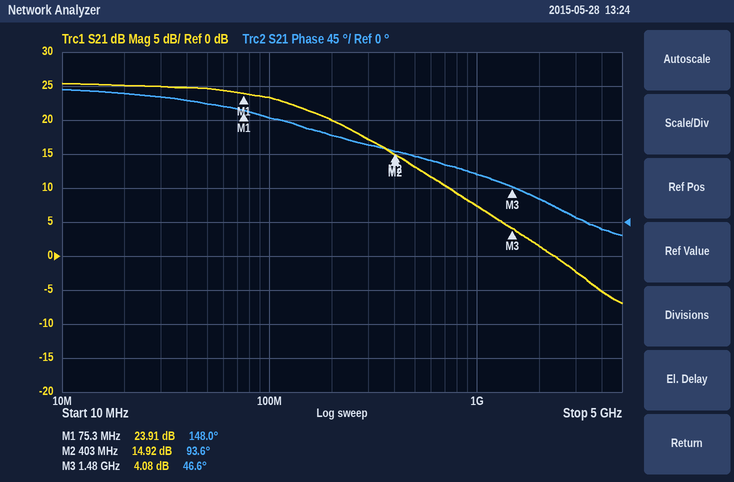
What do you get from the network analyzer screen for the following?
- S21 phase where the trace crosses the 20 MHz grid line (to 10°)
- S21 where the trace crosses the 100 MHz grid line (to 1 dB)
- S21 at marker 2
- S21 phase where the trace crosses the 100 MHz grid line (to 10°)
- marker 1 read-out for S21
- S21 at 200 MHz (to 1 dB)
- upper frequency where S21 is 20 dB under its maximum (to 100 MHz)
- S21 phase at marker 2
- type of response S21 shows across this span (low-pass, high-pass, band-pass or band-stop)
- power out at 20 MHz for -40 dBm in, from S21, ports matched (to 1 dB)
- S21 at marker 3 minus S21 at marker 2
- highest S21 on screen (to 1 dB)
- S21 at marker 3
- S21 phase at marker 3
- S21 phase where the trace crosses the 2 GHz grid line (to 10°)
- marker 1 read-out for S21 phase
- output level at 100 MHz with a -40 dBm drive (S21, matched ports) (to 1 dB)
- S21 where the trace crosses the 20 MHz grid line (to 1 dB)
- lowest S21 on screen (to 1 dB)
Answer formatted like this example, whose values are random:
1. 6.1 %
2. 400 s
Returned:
1. 170°
2. 23 dB
3. 14.92 dB
4. 140°
5. 23.91 dB
6. 20 dB
7. 1.3 GHz
8. 93.6°
9. low-pass
10. -15 dBm
11. -10.84 dB
12. 25 dB
13. 4.08 dB
14. 46.6°
15. 30°
16. 148.0°
17. -17 dBm
18. 25 dB
19. -7 dB
